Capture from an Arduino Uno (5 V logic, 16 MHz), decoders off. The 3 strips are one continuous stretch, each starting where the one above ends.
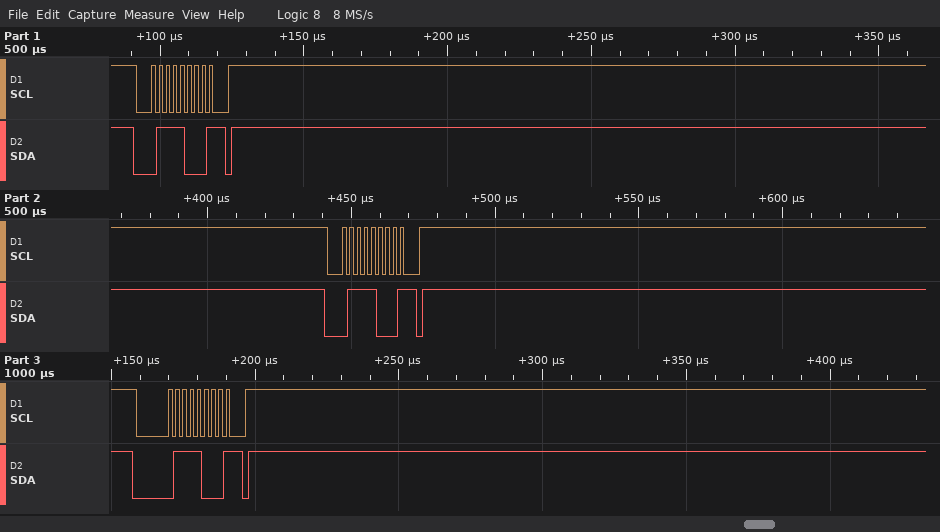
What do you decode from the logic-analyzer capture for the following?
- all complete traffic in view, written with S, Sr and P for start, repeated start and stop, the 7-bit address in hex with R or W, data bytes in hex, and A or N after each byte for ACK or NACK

S 3CW N P S 3CW N P S 3CW N P
